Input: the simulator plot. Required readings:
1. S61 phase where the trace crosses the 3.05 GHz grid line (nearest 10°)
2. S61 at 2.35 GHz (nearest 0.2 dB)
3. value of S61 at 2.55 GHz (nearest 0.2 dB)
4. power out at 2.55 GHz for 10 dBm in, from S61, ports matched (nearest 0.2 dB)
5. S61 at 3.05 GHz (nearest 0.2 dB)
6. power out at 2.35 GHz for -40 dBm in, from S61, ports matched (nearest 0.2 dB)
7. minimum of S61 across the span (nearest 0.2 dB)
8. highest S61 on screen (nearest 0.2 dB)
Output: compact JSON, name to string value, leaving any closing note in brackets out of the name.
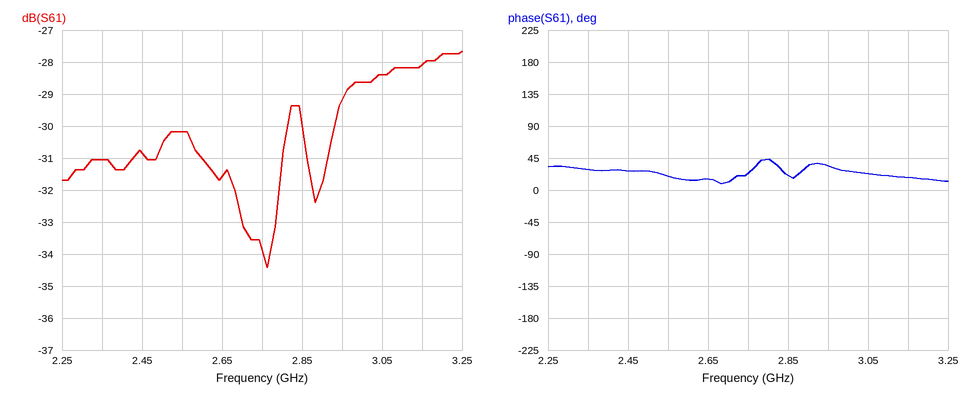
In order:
{"S61 phase where the trace crosses the 3.05 GHz grid line": "20°", "S61 at 2.35 GHz": "-31.0 dB", "value of S61 at 2.55 GHz": "-30.2 dB", "power out at 2.55 GHz for 10 dBm in, from S61, ports matched": "-20.2 dBm", "S61 at 3.05 GHz": "-28.4 dB", "power out at 2.35 GHz for -40 dBm in, from S61, ports matched": "-71.0 dBm", "minimum of S61 across the span": "-34.4 dB", "highest S61 on screen": "-27.6 dB"}
